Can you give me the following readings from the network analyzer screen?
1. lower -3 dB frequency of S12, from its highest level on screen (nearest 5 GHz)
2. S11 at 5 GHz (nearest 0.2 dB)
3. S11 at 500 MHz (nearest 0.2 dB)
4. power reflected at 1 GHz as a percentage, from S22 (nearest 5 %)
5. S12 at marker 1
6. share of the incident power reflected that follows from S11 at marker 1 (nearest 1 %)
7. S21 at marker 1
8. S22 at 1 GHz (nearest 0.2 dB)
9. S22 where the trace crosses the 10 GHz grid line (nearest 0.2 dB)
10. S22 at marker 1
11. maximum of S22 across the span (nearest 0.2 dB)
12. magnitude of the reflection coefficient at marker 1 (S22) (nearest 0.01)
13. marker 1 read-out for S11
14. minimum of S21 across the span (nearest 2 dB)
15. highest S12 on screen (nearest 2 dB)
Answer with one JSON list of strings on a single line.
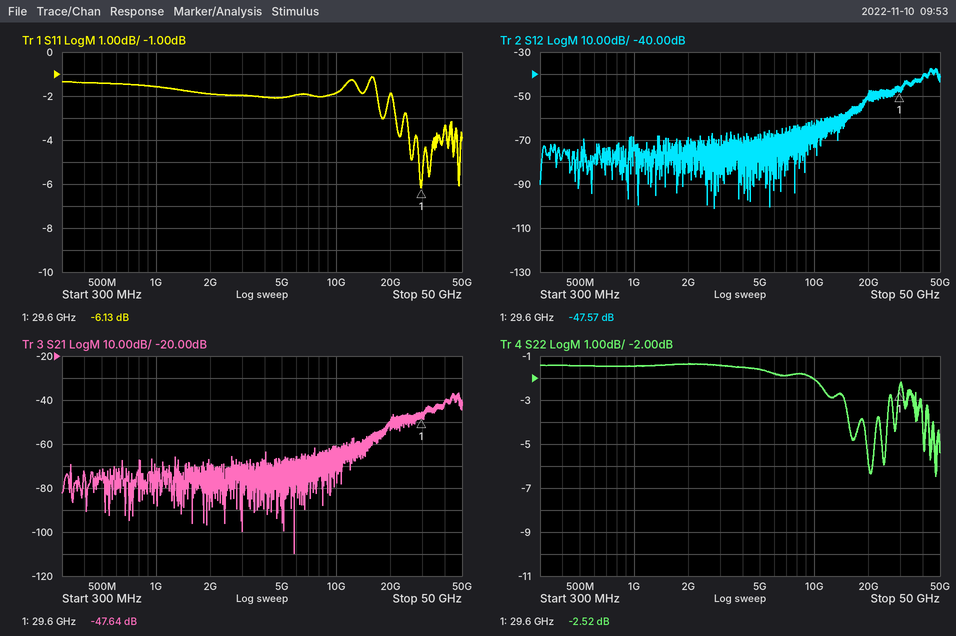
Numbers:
["45 GHz", "-2.0 dB", "-1.4 dB", "70 %", "-47.57 dB", "24 %", "-47.64 dB", "-1.4 dB", "-2.0 dB", "-2.52 dB", "-1.4 dB", "0.75", "-6.13 dB", "-110 dB", "-38 dB"]
